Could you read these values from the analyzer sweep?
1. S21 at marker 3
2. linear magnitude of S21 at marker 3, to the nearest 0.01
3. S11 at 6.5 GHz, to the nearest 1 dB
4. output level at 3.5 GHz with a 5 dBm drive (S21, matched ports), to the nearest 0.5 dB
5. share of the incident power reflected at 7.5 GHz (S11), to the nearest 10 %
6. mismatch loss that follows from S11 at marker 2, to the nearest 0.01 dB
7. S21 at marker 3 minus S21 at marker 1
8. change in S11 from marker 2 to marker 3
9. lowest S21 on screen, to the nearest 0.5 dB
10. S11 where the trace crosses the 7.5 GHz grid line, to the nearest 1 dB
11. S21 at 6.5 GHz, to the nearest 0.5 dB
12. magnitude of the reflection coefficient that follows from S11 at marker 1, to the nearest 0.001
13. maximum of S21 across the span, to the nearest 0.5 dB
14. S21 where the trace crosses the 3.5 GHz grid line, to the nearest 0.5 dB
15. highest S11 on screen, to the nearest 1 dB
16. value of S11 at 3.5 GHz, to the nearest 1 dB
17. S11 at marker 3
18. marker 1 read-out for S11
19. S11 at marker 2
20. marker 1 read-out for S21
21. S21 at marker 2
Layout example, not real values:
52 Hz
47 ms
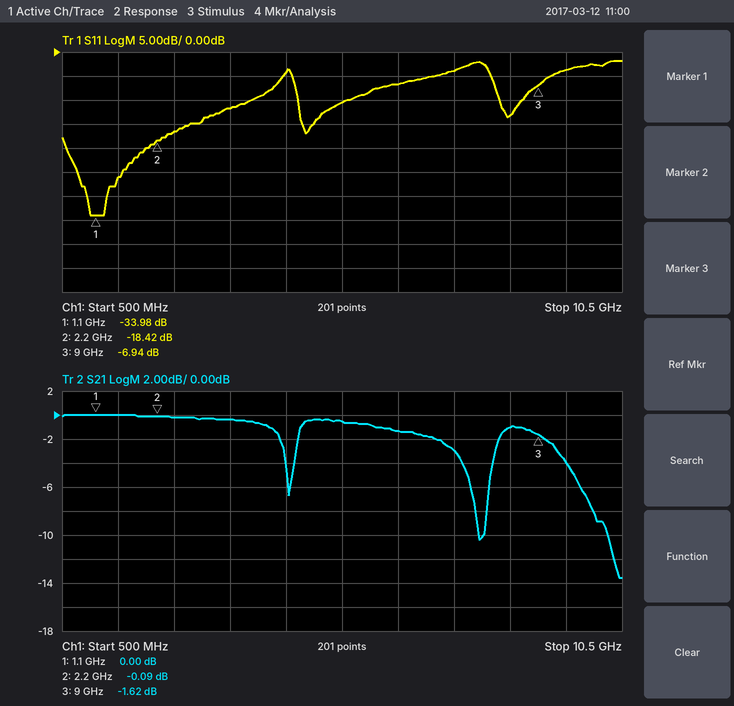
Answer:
-1.62 dB
0.83
-7 dB
4.5 dBm
40 %
0.06 dB
-1.62 dB
11.48 dB
-13.5 dB
-4 dB
-1.5 dB
0.020
0.0 dB
-0.5 dB
-2 dB
-12 dB
-6.94 dB
-33.98 dB
-18.42 dB
0.00 dB
-0.09 dB
